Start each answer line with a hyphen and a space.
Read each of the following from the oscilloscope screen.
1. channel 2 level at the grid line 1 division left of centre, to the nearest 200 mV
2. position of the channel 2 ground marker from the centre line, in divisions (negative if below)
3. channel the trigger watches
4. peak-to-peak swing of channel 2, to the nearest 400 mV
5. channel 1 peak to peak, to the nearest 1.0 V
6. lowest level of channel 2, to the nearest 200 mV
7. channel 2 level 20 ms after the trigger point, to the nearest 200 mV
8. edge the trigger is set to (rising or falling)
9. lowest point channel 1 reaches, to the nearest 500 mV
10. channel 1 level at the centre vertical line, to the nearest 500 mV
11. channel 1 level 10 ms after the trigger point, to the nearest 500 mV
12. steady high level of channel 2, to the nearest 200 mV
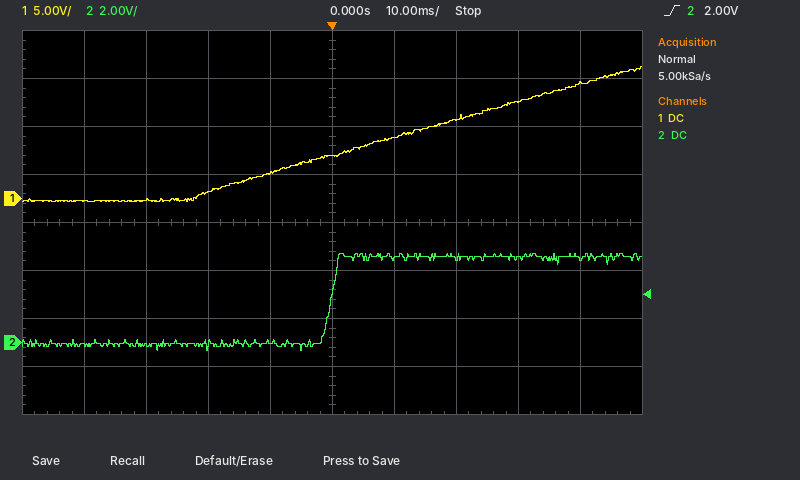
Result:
- 0.0 V
- -2.5 div
- channel 2
- 4.0 V
- 14.0 V
- -400 mV
- 3.6 V
- rising
- -500 mV
- 4.5 V
- 6.5 V
- 3.6 V
